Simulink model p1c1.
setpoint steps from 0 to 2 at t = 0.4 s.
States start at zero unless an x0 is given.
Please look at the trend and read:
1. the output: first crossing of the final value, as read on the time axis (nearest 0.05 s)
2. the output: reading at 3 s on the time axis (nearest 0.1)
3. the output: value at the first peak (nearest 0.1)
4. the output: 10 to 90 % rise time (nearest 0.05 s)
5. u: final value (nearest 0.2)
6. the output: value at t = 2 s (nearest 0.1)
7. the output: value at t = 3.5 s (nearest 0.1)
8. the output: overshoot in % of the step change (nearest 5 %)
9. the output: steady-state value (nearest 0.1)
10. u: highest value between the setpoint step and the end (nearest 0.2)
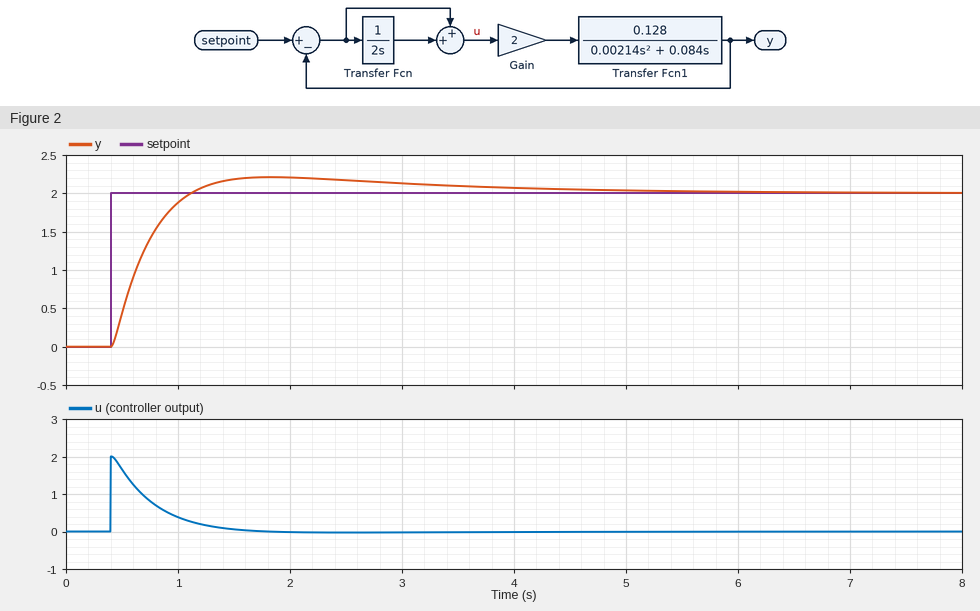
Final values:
1.10 s
2.1
2.2
0.50 s
0.0
2.2
2.1
10 %
2.0
2.0
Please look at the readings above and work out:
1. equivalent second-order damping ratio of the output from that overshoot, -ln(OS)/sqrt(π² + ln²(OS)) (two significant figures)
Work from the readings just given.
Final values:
0.59
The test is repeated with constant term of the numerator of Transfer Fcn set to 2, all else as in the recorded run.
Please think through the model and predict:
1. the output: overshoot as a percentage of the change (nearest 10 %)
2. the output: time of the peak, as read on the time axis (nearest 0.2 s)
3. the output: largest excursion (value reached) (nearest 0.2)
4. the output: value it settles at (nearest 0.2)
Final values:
20 %
1.6 s
2.4
2.0
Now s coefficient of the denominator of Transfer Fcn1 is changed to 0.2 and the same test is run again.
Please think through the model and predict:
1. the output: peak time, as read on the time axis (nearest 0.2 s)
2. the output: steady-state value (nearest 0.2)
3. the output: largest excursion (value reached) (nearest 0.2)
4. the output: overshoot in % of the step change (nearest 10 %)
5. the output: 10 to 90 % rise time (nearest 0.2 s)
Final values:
3.0 s
2.0
2.4
20 %
1.0 s
